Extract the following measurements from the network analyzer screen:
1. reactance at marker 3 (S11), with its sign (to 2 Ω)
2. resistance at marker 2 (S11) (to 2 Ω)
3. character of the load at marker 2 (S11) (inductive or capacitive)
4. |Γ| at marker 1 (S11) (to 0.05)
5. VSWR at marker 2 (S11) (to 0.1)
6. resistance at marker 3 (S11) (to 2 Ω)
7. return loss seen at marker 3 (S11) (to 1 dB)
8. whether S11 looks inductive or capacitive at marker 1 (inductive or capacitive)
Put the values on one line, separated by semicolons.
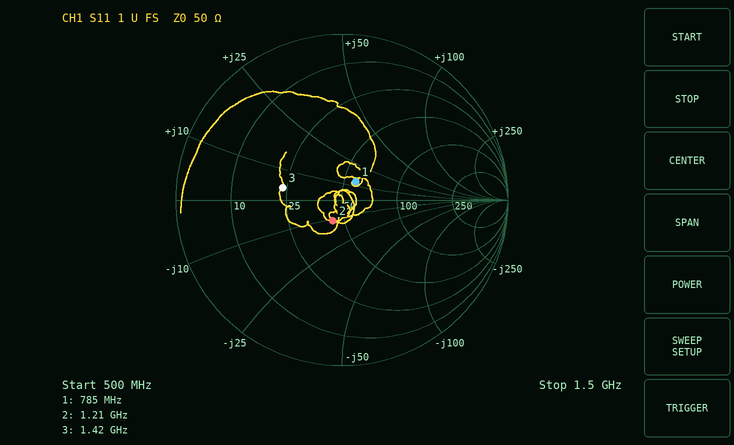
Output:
+4 Ω; 44 Ω; capacitive; 0.15; 1.3; 24 Ω; 9 dB; inductive
